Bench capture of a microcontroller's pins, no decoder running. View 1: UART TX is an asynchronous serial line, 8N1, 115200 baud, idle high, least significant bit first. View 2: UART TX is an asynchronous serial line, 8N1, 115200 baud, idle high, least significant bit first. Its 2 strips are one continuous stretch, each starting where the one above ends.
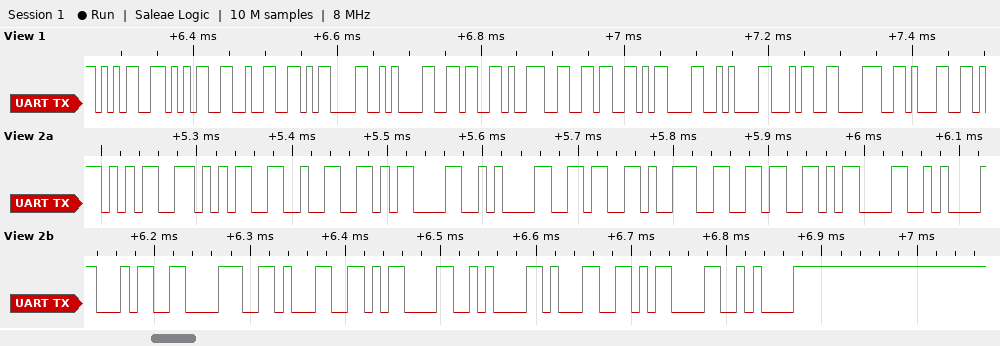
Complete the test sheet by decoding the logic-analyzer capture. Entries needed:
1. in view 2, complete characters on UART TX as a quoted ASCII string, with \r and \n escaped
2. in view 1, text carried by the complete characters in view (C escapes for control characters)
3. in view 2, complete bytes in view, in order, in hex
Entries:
"552\r\n696\r\n481\r\n1\r\n"
"552\r\n696\r\n481"
0x35 0x35 0x32 0x0D 0x0A 0x36 0x39 0x36 0x0D 0x0A 0x34 0x38 0x31 0x0D 0x0A 0x31 0x0D 0x0A
